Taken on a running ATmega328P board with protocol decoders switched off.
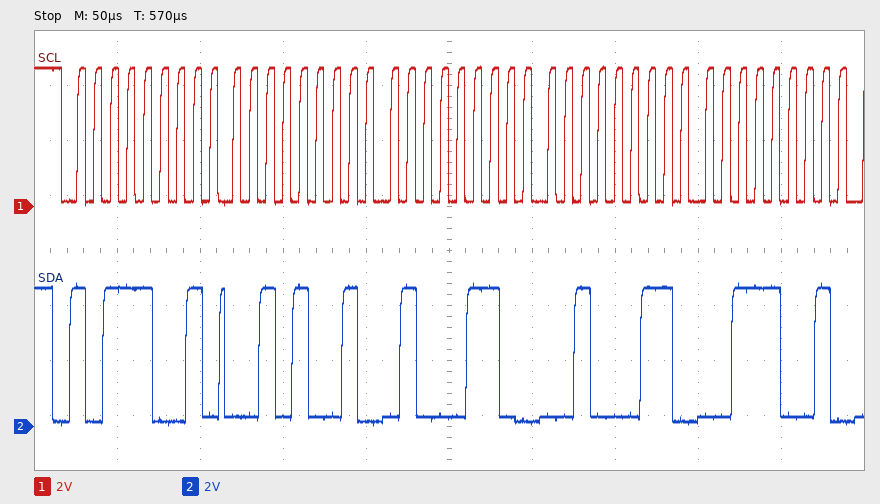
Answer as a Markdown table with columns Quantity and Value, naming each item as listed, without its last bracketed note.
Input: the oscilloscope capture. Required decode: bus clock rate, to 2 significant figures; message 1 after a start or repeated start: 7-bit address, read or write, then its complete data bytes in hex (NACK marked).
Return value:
| Quantity | Value |
|---|---|
| bus clock rate, to 2 significant figures | 100 kHz |
| message 1 after a start or repeated start: 7-bit address, read or write, then its complete data bytes in hex | 0x5C read: 29 46 23 39 |
